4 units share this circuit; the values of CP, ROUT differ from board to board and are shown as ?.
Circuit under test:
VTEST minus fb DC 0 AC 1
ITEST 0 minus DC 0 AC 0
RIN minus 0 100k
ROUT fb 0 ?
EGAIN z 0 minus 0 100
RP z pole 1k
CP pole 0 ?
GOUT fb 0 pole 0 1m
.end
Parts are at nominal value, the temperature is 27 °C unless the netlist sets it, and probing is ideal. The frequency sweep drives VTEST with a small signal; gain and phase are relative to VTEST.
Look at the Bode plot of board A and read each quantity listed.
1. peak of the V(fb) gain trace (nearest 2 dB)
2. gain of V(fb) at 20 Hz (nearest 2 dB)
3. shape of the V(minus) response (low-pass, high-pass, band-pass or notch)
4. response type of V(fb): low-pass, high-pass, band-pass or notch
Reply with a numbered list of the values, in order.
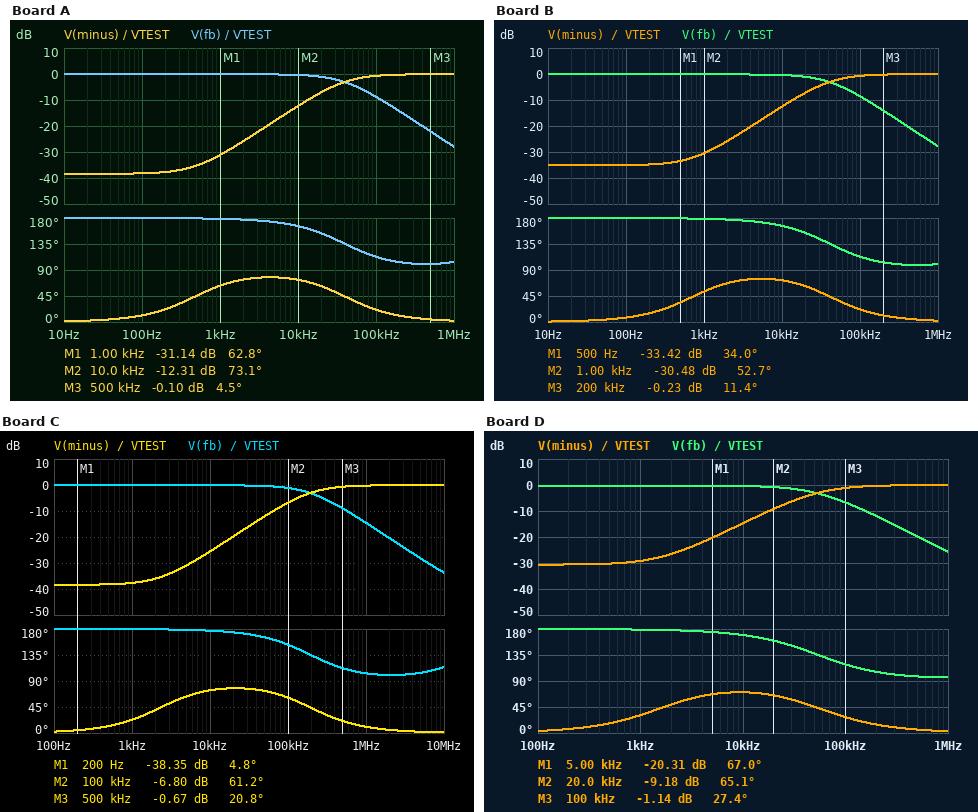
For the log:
1. 0 dB
2. 0 dB
3. high-pass
4. low-pass
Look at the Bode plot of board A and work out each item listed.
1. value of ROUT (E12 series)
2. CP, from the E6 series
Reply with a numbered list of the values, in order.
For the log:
1. 820 Ω
2. 330 nF
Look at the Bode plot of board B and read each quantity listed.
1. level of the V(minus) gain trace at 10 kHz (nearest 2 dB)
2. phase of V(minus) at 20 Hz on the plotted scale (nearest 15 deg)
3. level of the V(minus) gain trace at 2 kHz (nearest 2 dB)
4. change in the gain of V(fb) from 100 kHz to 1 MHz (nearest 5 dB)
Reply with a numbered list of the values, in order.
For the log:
1. -12 dB
2. 0 deg
3. -26 dB
4. -20 dB
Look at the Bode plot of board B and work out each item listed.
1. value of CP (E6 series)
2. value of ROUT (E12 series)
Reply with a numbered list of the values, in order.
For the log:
1. 220 nF
2. 560 Ω
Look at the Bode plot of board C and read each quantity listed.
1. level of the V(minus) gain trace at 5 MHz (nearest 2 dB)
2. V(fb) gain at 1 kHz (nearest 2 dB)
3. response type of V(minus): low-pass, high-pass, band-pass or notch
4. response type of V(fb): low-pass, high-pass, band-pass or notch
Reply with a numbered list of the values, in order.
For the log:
1. 0 dB
2. 0 dB
3. high-pass
4. low-pass
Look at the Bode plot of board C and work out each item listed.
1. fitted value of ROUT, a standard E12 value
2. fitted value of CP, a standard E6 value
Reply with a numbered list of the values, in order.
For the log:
1. 820 Ω
2. 68 nF
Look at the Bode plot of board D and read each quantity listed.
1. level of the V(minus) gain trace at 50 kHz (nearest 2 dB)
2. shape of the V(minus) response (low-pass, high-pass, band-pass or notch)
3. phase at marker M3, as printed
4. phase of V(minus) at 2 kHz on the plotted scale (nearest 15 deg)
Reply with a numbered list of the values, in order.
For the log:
1. -4 dB
2. high-pass
3. 27.4 deg
4. 45 deg
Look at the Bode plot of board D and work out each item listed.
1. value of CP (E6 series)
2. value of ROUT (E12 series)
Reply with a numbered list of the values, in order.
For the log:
1. 100 nF
2. 330 Ω
